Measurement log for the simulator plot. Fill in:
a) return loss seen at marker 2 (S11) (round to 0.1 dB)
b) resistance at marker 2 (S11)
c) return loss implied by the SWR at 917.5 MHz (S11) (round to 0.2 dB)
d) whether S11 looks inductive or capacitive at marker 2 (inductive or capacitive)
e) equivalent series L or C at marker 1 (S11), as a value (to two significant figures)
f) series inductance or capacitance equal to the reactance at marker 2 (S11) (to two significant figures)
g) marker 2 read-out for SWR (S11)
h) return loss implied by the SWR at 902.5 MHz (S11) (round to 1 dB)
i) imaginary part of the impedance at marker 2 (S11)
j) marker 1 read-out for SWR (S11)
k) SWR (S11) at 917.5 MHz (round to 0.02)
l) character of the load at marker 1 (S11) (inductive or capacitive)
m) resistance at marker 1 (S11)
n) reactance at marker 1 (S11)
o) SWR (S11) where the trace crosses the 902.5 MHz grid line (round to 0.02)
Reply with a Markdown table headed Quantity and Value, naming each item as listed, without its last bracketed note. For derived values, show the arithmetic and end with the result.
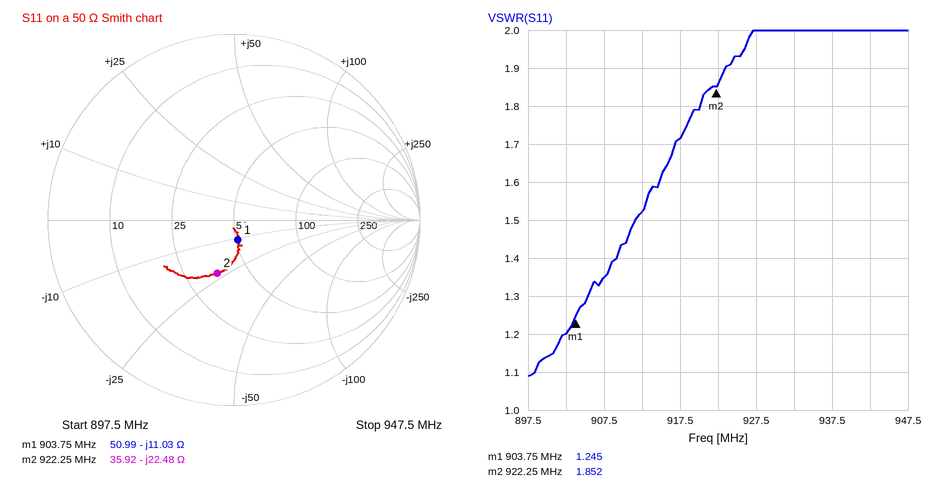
| Quantity | Value |
|---|---|
| return loss seen at marker 2 (S11) | 10.5 dB |
| resistance at marker 2 | 35.92 Ω |
| return loss implied by the SWR at 917.5 MHz (S11) | −20 log10((1.72 − 1)/(1.72 + 1)) ≈ 11.5 dB, so 11.6 dB to the nearest 0.2 dB |
| whether S11 looks inductive or capacitive at marker 2 | capacitive |
| equivalent series L or C at marker 1 (S11), as a value | C = 1/(2π × 903.75 MHz × 11.03 Ω) ≈ 16 pF |
| series inductance or capacitance equal to the reactance at marker 2 (S11) | C = 1/(2π × 922.25 MHz × 22.48 Ω) ≈ 7.7 pF |
| marker 2 read-out for SWR | 1.852 |
| return loss implied by the SWR at 902.5 MHz (S11) | −20 log10((1.2 − 1)/(1.2 + 1)) ≈ 21 dB |
| imaginary part of the impedance at marker 2 | -22.48 Ω |
| marker 1 read-out for SWR | 1.245 |
| SWR (S11) at 917.5 MHz | 1.72 |
| character of the load at marker 1 (S11) | capacitive |
| resistance at marker 1 | 50.99 Ω |
| reactance at marker 1 | -11.03 Ω |
| SWR (S11) where the trace crosses the 902.5 MHz grid line | 1.20 |
